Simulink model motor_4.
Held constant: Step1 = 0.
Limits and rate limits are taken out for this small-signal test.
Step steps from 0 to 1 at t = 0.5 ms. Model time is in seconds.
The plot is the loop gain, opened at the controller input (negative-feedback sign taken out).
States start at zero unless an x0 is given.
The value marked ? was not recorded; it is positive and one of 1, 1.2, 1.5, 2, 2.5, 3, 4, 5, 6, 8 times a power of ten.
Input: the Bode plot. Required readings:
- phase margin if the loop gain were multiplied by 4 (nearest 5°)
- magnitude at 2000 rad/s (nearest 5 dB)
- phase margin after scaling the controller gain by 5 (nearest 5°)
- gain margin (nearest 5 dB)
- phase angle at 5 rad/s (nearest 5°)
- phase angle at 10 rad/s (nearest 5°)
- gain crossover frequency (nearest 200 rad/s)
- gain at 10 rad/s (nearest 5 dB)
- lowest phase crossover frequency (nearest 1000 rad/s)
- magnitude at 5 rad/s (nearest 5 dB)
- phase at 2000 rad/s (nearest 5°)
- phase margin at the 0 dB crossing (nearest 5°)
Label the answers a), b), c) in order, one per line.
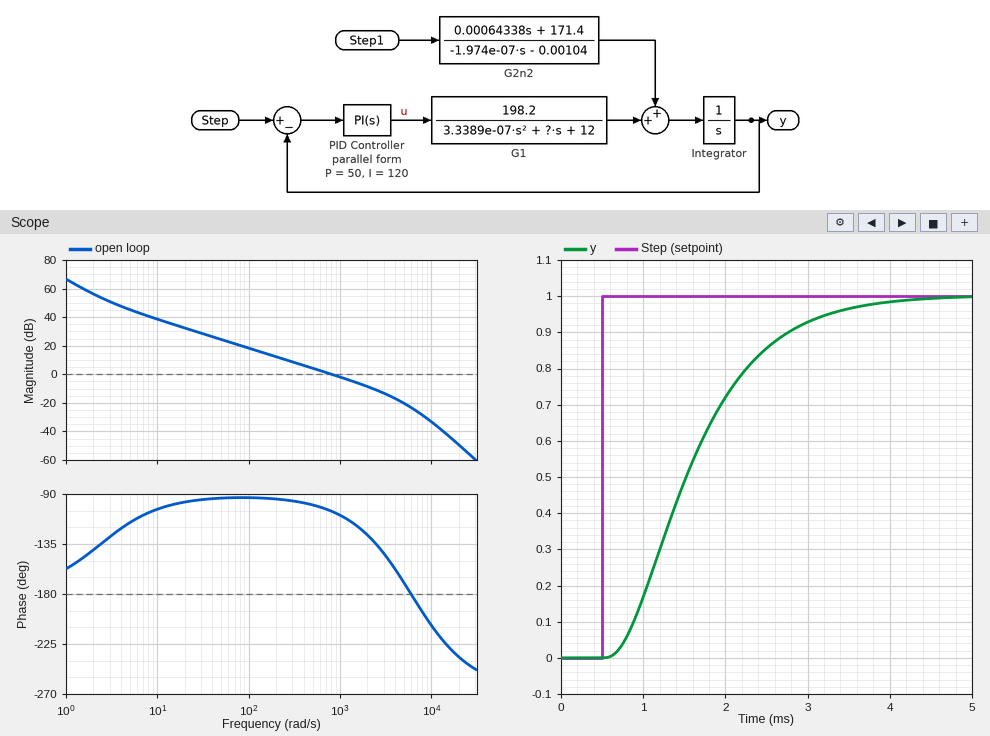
a) 40°
b) -10 dB
c) 35°
d) 25 dB
e) -115°
f) -105°
g) 800 rad/s
h) 40 dB
i) 6000 rad/s
j) 45 dB
k) -125°
l) 75°
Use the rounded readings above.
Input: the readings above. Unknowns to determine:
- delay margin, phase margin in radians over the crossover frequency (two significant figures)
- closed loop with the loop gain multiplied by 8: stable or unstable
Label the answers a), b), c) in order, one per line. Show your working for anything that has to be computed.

a) 75 × π / 180 / 800 = 0.0016 s
b) stable
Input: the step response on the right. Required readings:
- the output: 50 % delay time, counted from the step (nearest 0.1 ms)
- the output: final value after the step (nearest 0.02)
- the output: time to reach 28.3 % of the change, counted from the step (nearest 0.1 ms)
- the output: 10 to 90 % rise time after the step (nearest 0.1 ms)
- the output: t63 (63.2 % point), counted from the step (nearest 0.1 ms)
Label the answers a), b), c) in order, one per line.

a) 1.0 ms
b) 1.00
c) 0.7 ms
d) 1.9 ms
e) 1.3 ms
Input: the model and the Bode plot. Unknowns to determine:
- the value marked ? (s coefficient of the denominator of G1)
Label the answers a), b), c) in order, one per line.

a) 0.004
